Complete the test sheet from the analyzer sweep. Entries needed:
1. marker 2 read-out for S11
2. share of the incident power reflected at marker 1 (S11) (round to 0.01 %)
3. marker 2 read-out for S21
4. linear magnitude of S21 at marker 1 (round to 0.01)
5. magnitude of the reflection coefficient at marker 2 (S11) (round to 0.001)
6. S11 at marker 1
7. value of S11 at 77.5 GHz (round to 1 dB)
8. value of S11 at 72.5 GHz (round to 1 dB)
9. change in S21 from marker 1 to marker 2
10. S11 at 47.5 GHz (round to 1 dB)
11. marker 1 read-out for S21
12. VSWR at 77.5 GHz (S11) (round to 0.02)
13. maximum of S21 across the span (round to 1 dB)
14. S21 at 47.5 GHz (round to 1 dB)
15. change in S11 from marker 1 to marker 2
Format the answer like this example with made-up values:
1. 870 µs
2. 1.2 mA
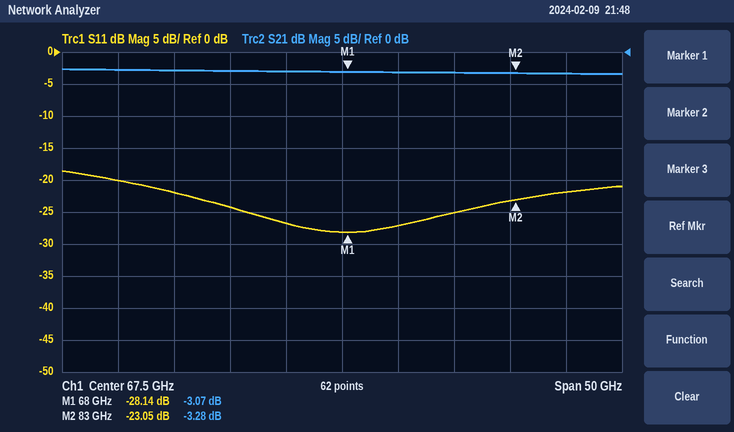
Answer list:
1. -23.05 dB
2. 0.15 %
3. -3.28 dB
4. 0.70
5. 0.070
6. -28.14 dB
7. -25 dB
8. -27 dB
9. -0.21 dB
10. -20 dB
11. -3.07 dB
12. 1.12
13. -3 dB
14. -3 dB
15. 5.09 dB
